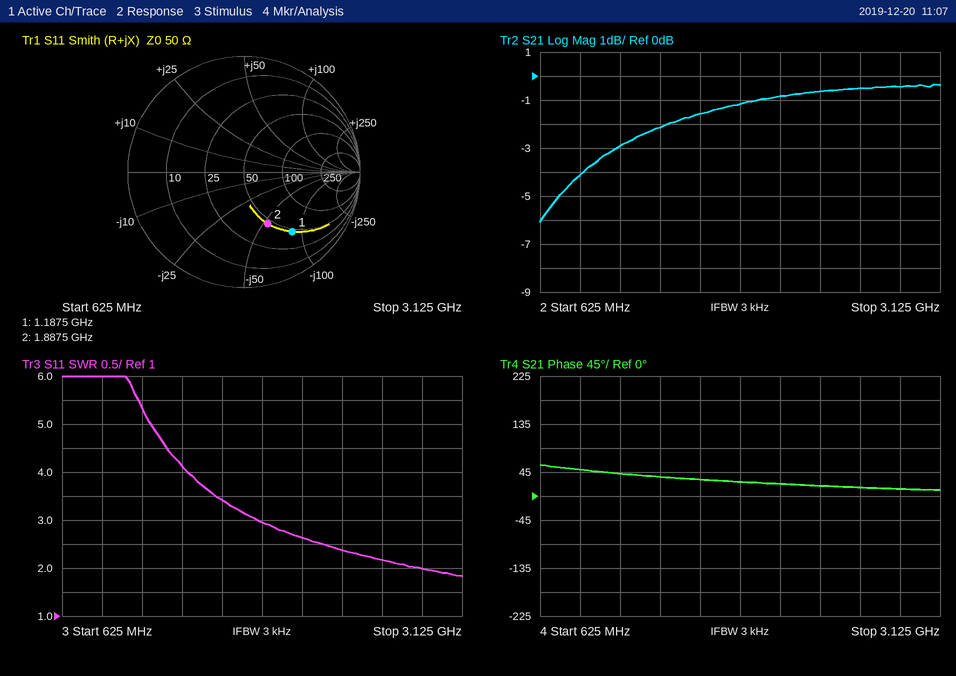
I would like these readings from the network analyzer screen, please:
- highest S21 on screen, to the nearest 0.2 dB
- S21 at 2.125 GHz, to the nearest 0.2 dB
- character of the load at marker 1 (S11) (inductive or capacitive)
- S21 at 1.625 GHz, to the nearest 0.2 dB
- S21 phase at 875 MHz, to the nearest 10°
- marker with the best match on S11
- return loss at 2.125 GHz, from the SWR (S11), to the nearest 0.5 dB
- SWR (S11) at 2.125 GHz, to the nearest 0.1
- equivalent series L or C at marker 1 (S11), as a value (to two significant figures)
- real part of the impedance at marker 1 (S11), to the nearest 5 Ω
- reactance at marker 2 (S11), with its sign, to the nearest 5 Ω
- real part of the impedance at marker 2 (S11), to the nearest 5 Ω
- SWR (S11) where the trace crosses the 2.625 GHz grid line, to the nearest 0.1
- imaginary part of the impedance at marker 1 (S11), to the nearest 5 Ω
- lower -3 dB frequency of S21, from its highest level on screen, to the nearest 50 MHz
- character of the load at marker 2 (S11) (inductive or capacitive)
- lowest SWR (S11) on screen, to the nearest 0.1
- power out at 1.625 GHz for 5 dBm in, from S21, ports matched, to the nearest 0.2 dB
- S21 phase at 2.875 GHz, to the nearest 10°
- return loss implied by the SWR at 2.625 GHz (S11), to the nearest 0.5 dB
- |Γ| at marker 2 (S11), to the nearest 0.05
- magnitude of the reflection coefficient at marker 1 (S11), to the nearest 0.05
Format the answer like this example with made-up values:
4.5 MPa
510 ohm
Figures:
-0.4 dB
-0.8 dB
capacitive
-1.6 dB
50°
marker 2
7.0 dB
2.6
1.6 pF
45 Ω
-55 Ω
45 Ω
2.2
-85 Ω
1.00 GHz
capacitive
1.8
3.4 dBm
10°
8.5 dB
0.50
0.65
